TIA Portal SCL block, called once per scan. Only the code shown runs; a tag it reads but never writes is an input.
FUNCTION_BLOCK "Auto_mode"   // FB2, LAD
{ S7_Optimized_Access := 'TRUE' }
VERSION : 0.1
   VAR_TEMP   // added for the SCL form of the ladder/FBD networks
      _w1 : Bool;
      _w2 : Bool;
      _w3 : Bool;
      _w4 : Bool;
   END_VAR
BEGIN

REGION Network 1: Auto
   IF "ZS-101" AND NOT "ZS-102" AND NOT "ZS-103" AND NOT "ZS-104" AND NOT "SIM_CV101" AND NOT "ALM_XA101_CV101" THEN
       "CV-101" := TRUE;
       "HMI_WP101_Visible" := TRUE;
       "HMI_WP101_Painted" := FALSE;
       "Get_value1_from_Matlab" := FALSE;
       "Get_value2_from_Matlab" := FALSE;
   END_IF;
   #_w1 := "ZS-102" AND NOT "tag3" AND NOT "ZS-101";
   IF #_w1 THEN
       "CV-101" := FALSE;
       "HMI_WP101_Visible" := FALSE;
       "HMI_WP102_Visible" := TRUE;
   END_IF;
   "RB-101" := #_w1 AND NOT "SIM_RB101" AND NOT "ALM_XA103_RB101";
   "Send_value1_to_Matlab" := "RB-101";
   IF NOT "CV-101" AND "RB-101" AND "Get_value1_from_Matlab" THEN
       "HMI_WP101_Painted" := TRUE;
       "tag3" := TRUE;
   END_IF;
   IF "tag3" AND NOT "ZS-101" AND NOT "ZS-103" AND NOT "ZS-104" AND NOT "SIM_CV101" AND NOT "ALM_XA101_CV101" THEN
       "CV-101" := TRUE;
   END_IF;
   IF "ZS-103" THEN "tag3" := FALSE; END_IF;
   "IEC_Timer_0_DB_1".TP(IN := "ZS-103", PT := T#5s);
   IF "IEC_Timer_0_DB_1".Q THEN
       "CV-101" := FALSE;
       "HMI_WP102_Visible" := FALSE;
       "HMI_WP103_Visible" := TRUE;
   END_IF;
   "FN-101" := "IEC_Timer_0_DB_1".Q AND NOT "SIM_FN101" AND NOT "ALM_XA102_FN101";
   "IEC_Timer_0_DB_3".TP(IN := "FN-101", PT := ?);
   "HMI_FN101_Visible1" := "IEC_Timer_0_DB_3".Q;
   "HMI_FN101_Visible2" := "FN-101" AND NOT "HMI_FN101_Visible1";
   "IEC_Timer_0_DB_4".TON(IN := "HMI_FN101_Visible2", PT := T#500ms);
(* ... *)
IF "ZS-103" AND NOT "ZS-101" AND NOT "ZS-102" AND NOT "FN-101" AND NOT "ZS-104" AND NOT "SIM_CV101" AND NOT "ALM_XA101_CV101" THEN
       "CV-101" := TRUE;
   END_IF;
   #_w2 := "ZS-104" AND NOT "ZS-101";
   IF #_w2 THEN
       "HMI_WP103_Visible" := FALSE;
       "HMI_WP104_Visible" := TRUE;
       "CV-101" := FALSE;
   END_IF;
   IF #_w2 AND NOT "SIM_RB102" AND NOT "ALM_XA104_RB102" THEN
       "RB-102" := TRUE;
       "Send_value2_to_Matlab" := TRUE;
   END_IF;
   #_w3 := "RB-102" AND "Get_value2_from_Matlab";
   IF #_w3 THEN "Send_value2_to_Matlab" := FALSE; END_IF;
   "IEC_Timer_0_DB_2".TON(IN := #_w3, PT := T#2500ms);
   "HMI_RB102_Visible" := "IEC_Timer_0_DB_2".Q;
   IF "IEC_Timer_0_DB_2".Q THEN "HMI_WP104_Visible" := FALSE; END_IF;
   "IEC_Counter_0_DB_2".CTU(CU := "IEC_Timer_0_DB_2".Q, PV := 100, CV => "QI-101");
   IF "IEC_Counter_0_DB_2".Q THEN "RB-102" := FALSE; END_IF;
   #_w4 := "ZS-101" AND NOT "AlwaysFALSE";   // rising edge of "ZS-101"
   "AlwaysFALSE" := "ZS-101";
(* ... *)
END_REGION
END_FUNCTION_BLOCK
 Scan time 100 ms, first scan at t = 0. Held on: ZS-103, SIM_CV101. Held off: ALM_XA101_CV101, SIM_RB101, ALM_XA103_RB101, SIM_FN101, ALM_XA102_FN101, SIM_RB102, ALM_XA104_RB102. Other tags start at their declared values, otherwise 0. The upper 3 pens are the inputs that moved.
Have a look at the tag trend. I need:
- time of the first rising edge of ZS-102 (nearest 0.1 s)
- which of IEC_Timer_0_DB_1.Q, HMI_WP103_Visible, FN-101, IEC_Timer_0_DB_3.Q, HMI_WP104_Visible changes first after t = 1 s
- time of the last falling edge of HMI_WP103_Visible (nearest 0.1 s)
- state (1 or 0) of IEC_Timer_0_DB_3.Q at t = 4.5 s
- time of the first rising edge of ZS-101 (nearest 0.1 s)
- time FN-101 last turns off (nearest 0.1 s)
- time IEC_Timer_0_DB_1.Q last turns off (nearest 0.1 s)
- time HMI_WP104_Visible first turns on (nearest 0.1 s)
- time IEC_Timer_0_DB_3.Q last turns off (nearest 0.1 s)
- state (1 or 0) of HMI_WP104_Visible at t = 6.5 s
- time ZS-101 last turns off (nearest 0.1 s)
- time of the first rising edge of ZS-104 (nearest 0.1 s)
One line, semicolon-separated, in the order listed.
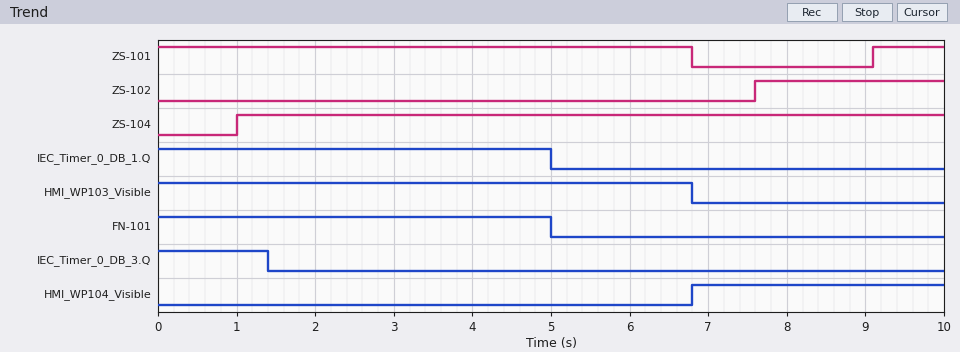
7.6 s; IEC_Timer_0_DB_3.Q; 6.8 s; 0; 9.1 s; 5.0 s; 5.0 s; 6.8 s; 1.4 s; 0; 6.8 s; 1.0 s
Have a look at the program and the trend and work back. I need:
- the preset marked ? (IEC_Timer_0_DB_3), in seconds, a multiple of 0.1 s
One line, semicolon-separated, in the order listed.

1.4 s
